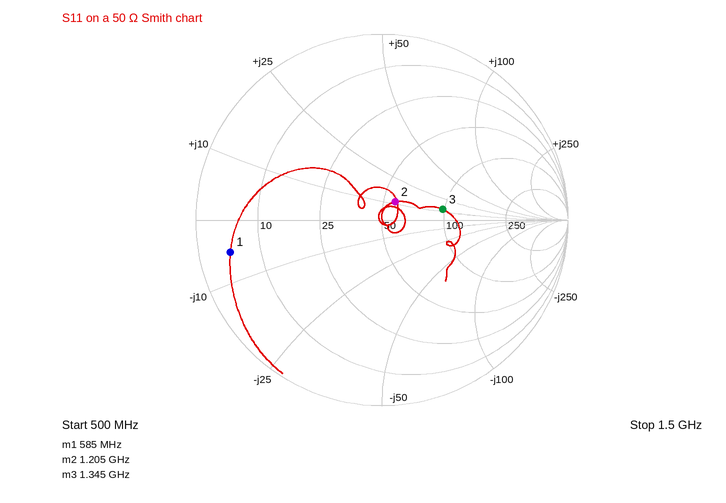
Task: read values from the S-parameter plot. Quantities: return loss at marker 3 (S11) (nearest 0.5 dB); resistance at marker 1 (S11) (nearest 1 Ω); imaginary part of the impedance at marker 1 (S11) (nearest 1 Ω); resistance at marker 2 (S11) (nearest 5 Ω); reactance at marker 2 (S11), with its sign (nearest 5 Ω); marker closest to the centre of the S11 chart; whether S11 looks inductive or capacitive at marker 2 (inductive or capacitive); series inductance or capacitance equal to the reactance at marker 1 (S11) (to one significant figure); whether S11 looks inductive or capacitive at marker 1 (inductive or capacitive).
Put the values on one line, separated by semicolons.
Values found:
9.5 dB; 5 Ω; -5 Ω; 55 Ω; +10 Ω; marker 2; inductive; 50 pF; capacitive
